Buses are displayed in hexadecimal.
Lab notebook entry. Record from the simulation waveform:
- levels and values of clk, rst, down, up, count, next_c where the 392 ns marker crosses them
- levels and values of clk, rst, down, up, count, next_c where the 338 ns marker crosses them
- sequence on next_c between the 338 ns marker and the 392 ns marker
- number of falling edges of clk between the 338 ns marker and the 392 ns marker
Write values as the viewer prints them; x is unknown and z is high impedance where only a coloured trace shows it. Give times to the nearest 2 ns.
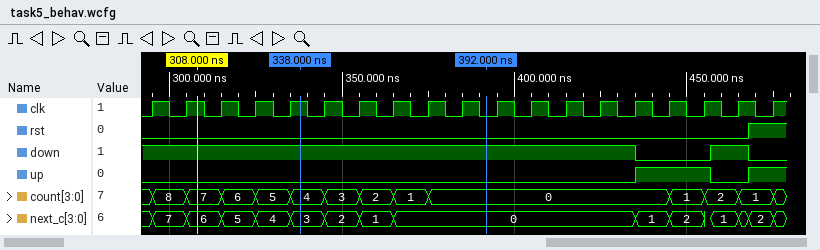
clk=0, rst=0, down=1, up=0, count=0, next_c=0
clk=1, rst=0, down=1, up=0, count=4, next_c=3
3, 2, 1, 0
6
